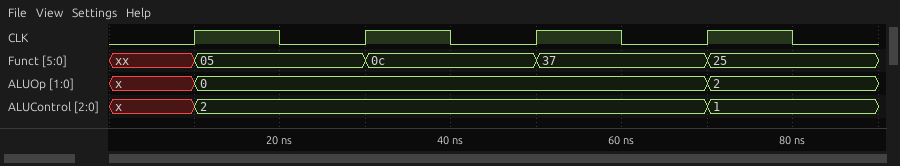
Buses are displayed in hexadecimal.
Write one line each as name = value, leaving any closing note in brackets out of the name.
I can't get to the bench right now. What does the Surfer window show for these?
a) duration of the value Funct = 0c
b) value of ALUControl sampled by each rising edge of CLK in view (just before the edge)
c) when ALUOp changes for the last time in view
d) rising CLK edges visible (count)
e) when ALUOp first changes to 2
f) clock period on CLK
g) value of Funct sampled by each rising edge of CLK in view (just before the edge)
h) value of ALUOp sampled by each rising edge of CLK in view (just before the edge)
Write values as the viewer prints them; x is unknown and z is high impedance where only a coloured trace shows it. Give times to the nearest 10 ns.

duration of the value Funct = 0c = 20 ns
value of ALUControl sampled by each rising edge of CLK in view = x, 2, 2, 2
when ALUOp changes for the last time in view = 70 ns
rising CLK edges visible = 4
when ALUOp first changes to 2 = 70 ns
clock period on CLK = 20 ns
value of Funct sampled by each rising edge of CLK in view = xx, 05, 0c, 37
value of ALUOp sampled by each rising edge of CLK in view = x, 0, 0, 0
